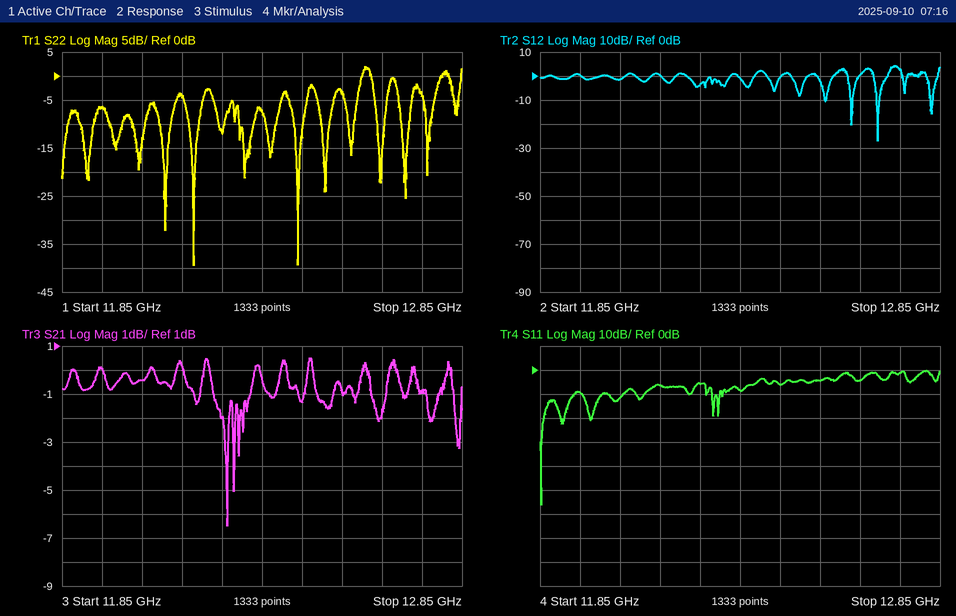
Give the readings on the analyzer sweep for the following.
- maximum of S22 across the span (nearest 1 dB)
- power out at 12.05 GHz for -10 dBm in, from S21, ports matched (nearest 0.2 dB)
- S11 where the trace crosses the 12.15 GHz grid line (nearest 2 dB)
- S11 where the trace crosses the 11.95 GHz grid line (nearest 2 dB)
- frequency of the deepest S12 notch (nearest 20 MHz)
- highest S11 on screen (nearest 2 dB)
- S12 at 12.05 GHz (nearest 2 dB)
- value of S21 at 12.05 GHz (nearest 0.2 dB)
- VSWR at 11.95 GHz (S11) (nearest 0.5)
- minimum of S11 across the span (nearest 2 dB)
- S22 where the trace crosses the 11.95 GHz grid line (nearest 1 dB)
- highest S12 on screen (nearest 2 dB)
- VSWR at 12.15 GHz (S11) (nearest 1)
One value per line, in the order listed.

2 dB
-10.4 dBm
-6 dB
-10 dB
12.70 GHz
0 dB
-2 dB
-0.4 dB
2.0
-56 dB
-7 dB
4 dB
3
